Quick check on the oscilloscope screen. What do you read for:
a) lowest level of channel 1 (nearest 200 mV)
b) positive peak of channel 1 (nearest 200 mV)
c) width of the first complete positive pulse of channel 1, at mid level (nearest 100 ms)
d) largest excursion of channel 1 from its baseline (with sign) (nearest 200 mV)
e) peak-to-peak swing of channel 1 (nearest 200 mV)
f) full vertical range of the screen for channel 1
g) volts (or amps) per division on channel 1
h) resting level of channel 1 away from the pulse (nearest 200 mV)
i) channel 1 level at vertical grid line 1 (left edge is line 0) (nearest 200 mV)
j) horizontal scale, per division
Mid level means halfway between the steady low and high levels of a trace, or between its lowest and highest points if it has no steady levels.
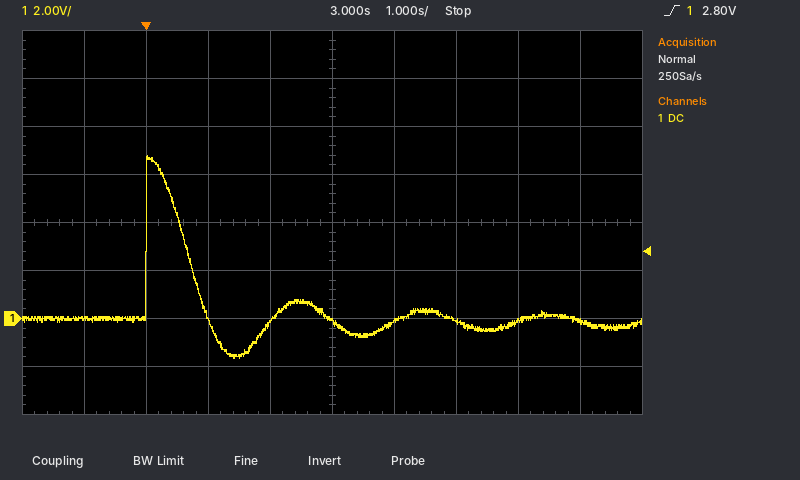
-1.6 V
6.8 V
700 ms
+6.8 V
8.4 V
16 V
2 V
0.0 V
0.0 V
1 s
